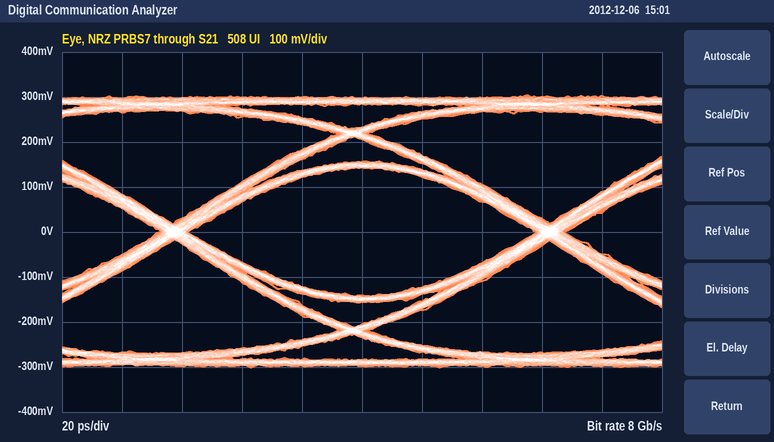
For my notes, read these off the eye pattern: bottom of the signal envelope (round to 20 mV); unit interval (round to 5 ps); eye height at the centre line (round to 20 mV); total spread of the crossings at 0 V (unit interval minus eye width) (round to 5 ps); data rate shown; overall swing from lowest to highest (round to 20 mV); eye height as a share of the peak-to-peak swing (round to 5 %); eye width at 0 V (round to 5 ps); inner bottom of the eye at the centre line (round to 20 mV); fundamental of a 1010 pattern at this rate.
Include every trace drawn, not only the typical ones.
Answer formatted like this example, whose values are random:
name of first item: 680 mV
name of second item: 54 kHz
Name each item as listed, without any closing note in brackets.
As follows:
bottom of the signal envelope: -300 mV
unit interval: 125 ps
eye height at the centre line: 280 mV
total spread of the crossings at 0 V (unit interval minus eye width): 10 ps
data rate shown: 8 Gb/s
overall swing from lowest to highest: 600 mV
eye height as a share of the peak-to-peak swing: 45 %
eye width at 0 V: 115 ps
inner bottom of the eye at the centre line: -140 mV
fundamental of a 1010 pattern at this rate: 4 GHz
